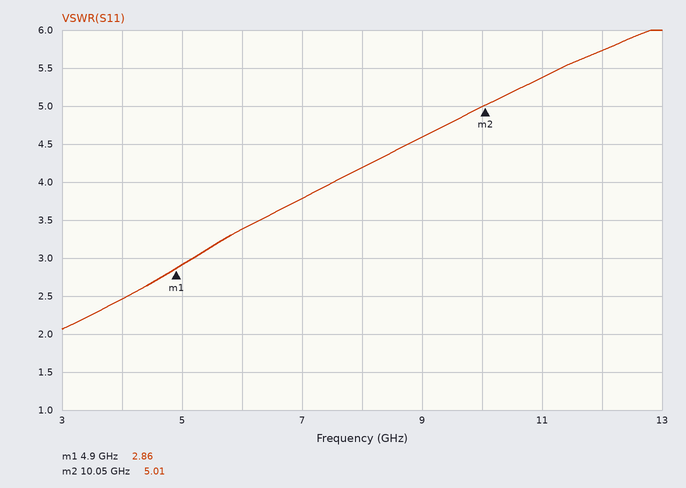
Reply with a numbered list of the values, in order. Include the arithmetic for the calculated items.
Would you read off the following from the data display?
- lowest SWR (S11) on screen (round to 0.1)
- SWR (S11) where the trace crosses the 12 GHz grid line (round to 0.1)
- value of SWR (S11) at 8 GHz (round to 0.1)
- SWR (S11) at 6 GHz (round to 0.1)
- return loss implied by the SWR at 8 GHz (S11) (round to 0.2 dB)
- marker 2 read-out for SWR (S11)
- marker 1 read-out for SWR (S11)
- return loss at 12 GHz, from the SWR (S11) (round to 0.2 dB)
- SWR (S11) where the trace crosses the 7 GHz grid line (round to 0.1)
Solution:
1. 2.1
2. 5.7
3. 4.2
4. 3.4
5. −20 log10((4.2 − 1)/(4.2 + 1)) ≈ 4.2 dB
6. 5.01
7. 2.86
8. −20 log10((5.7 − 1)/(5.7 + 1)) ≈ 3.08 dB, so 3.0 dB to the nearest 0.2 dB
9. 3.8
